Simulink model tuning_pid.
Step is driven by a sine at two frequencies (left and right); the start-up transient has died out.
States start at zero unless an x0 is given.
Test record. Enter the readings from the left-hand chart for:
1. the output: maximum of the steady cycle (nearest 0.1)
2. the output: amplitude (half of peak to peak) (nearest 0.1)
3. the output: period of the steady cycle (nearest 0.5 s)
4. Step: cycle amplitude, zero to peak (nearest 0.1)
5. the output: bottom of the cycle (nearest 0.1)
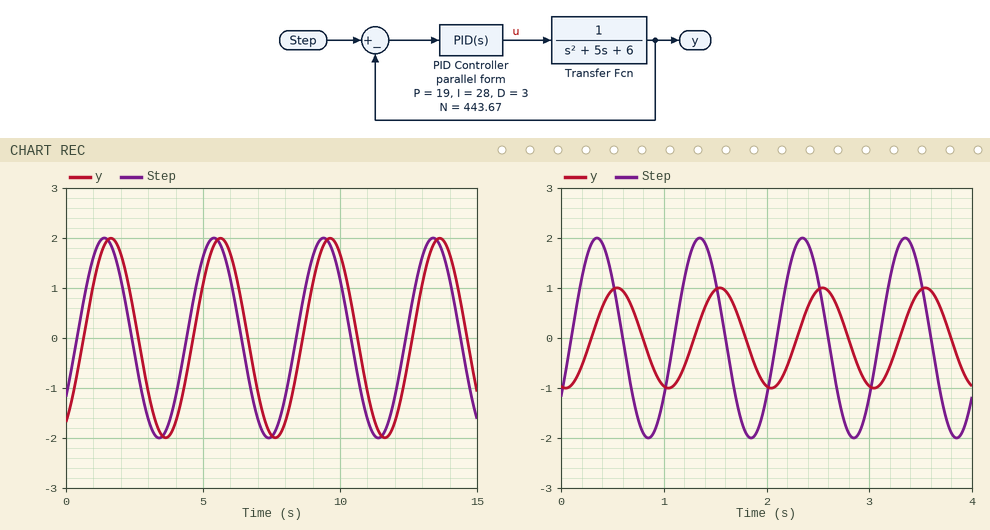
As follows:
2.0
2.0
4.0 s
2.0
-2.0
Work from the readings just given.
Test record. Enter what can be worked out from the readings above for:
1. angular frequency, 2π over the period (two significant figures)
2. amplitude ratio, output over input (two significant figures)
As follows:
1.6 rad/s
1.0
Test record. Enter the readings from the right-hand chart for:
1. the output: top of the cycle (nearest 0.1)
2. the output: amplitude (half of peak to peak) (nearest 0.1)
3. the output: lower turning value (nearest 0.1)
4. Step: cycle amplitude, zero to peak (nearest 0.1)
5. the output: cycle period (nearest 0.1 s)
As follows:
1.0
1.0
-1.0
2.0
1.0 s
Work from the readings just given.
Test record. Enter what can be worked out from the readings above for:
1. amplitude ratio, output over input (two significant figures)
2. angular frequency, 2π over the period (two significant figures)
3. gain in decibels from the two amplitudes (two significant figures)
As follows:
0.50
6.3 rad/s
-6.0 dB
